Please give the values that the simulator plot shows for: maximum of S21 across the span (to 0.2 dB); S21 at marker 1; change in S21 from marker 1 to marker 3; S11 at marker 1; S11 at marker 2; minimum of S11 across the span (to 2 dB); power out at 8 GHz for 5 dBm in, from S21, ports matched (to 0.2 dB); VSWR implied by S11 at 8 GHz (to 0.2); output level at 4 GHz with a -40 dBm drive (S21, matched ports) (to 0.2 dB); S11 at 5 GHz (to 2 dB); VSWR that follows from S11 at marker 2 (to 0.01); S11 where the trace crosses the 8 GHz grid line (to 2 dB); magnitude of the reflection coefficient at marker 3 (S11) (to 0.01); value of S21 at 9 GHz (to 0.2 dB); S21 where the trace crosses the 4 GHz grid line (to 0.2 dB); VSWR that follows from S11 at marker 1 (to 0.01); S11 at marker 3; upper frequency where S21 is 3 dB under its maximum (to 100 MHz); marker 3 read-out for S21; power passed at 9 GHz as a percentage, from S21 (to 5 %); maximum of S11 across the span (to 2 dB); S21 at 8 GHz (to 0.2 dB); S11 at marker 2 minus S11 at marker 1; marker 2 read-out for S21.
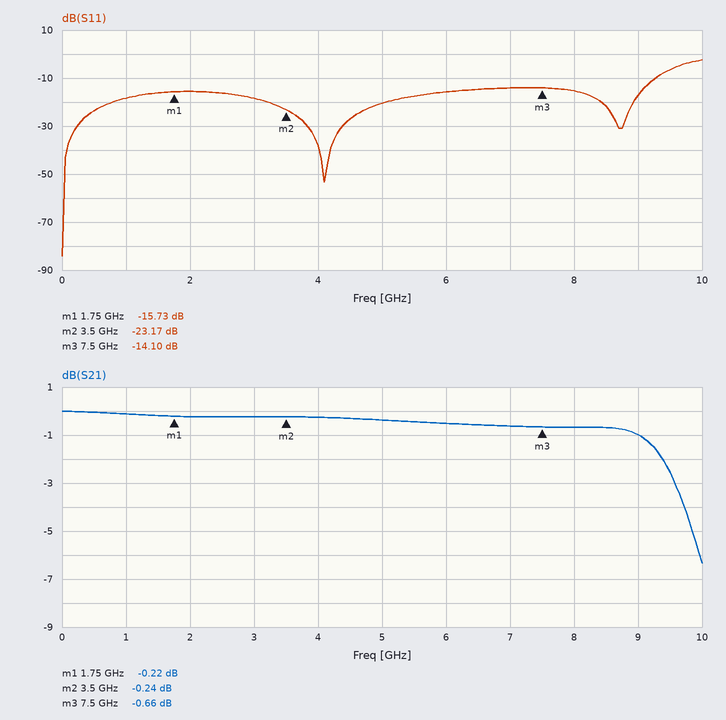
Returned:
0.0 dB
-0.22 dB
-0.44 dB
-15.73 dB
-23.17 dB
-84 dB
4.4 dBm
1.4
-40.2 dBm
-20 dB
1.15
-16 dB
0.20
-1.0 dB
-0.2 dB
1.39
-14.10 dB
9.6 GHz
-0.66 dB
80 %
-2 dB
-0.6 dB
-7.44 dB
-0.24 dB
